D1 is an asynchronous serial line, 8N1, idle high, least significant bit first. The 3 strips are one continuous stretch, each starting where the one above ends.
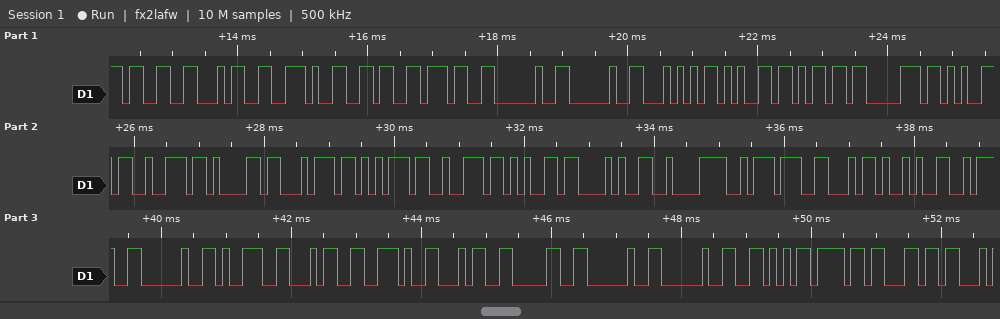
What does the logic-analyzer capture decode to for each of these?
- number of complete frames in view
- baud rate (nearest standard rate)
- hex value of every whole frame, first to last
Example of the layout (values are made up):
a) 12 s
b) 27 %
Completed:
a) 35
b) 9600 baud
c) 33 34 2E 36 37 20 20 54 65 6D 70 65 72 61 74 75 72 65 28 C2 BA 46 29 3A 20 39 34 2E 34 30 20 20 56 6F 6C
